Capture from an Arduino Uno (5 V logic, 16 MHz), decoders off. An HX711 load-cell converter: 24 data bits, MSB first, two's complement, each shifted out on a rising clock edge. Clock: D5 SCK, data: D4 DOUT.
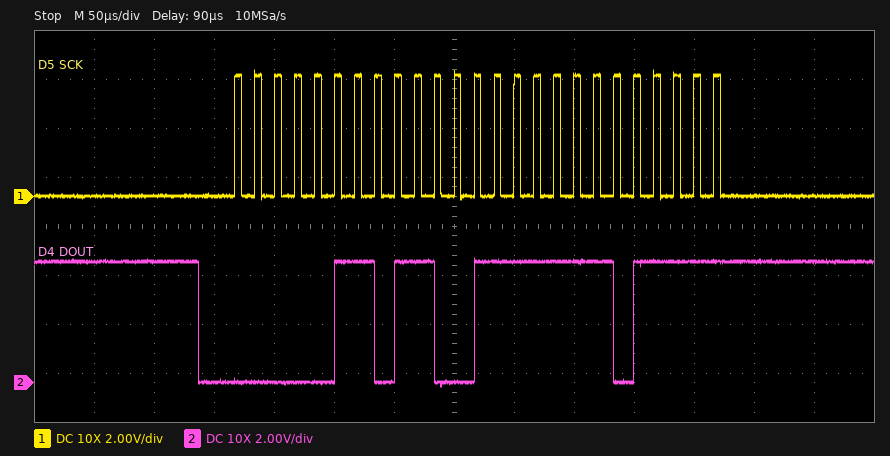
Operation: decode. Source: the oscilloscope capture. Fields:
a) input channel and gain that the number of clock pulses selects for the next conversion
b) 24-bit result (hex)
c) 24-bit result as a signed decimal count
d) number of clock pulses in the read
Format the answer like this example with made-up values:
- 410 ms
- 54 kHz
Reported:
- channel A, gain 128
- 0x06CFEF
- 446447
- 25
